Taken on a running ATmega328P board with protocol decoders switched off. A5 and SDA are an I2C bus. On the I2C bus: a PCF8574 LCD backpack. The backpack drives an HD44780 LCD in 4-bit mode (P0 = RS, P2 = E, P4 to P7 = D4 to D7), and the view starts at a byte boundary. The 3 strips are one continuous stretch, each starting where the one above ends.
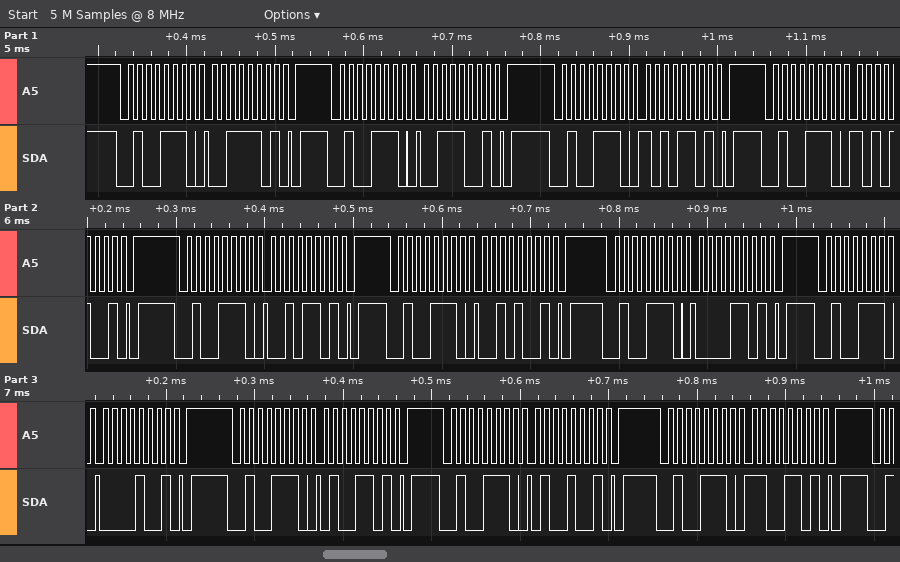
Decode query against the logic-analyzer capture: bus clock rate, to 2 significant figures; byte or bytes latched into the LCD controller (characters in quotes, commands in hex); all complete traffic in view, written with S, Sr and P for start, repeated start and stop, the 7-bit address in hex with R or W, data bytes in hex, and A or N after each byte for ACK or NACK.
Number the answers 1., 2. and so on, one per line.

1. 100 kHz
2. ':' ' '
3. S 27W A 3D A P S 27W A 39 A P S 27W A AD A P S 27W A A9 A P S 27W A 2D A P S 27W A 29 A P S 27W A 0D A P S 27W A 09 A P S 27W A 4D A P S 27W A 49 A P S 27W A CD A P
